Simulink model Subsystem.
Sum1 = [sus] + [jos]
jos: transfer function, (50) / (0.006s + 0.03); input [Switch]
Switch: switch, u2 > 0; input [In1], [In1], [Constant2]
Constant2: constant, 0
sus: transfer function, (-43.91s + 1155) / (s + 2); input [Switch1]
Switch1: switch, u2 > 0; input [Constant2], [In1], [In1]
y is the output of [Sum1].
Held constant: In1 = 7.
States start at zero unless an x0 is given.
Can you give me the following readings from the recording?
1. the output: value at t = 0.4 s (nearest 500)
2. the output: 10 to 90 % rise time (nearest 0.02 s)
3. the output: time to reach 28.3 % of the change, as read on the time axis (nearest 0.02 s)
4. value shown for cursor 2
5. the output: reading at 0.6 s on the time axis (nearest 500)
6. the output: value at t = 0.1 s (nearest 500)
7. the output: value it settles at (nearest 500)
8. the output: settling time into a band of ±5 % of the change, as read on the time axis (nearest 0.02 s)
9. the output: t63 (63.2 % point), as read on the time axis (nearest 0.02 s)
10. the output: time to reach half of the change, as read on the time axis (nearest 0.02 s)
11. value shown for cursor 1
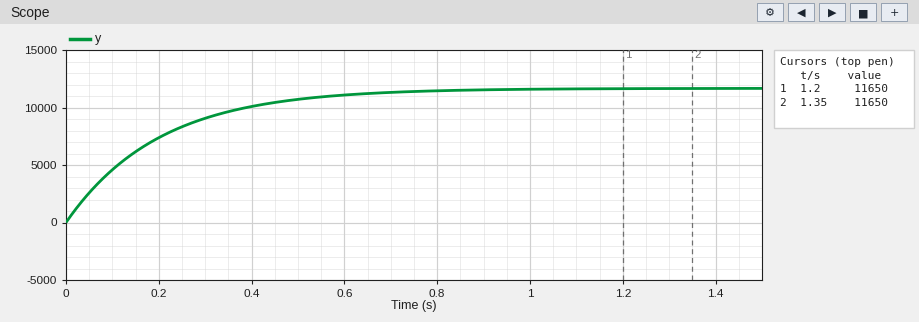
10000
0.44 s
0.06 s
11650
11000
4500
11500
0.60 s
0.20 s
0.14 s
11650
